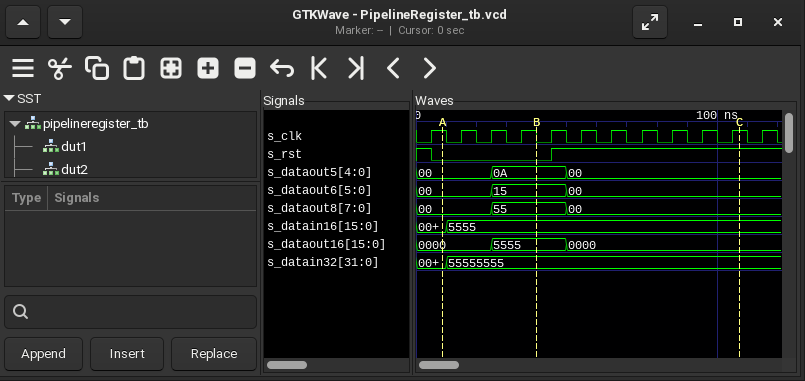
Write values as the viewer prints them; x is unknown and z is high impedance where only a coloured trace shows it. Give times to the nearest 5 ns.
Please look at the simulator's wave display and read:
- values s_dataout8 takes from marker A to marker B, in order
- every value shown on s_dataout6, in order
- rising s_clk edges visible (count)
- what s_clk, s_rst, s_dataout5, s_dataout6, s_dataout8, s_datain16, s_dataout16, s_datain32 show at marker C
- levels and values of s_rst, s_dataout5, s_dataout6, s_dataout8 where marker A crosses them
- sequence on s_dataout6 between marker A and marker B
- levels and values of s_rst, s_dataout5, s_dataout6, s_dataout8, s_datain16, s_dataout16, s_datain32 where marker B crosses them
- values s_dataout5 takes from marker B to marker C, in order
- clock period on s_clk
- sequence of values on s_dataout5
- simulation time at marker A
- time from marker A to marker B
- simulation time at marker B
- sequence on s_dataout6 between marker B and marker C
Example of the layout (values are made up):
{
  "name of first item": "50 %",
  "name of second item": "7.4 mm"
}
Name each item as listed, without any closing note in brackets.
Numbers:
{
  "values s_dataout8 takes from marker A to marker B, in order": "00, 55",
  "every value shown on s_dataout6, in order": "00, 15, 00",
  "rising s_clk edges visible": "12",
  "what s_clk, s_rst, s_dataout5, s_dataout6, s_dataout8, s_datain16, s_dataout16, s_datain32 show at marker C": "s_clk=1, s_rst=1, s_dataout5=00, s_dataout6=00, s_dataout8=00, s_datain16=5555, s_dataout16=0000, s_datain32=55555555",
  "levels and values of s_rst, s_dataout5, s_dataout6, s_dataout8 where marker A crosses them": "s_rst=0, s_dataout5=00, s_dataout6=00, s_dataout8=00",
  "sequence on s_dataout6 between marker A and marker B": "00, 15",
  "levels and values of s_rst, s_dataout5, s_dataout6, s_dataout8, s_datain16, s_dataout16, s_datain32 where marker B crosses them": "s_rst=0, s_dataout5=0A, s_dataout6=15, s_dataout8=55, s_datain16=5555, s_dataout16=5555, s_datain32=55555555",
  "values s_dataout5 takes from marker B to marker C, in order": "0A, 00",
  "clock period on s_clk": "10 ns",
  "sequence of values on s_dataout5": "00, 0A, 00",
  "simulation time at marker A": "10 ns",
  "time from marker A to marker B": "30 ns",
  "simulation time at marker B": "40 ns",
  "sequence on s_dataout6 between marker B and marker C": "15, 00"
}
